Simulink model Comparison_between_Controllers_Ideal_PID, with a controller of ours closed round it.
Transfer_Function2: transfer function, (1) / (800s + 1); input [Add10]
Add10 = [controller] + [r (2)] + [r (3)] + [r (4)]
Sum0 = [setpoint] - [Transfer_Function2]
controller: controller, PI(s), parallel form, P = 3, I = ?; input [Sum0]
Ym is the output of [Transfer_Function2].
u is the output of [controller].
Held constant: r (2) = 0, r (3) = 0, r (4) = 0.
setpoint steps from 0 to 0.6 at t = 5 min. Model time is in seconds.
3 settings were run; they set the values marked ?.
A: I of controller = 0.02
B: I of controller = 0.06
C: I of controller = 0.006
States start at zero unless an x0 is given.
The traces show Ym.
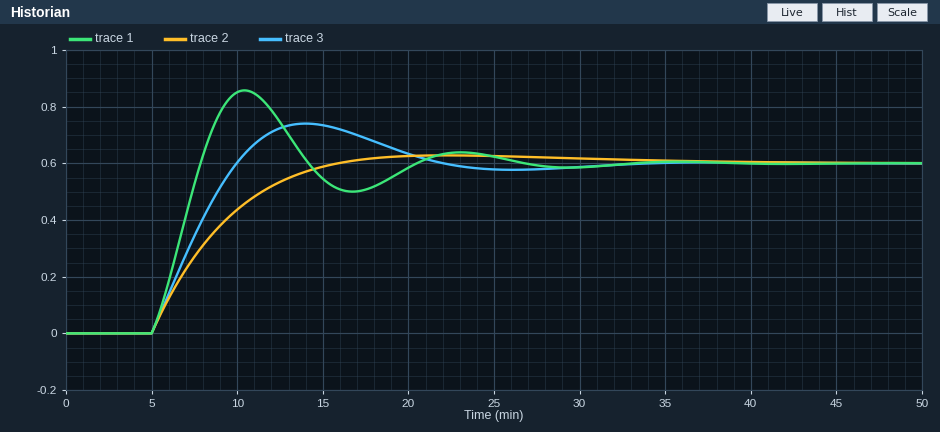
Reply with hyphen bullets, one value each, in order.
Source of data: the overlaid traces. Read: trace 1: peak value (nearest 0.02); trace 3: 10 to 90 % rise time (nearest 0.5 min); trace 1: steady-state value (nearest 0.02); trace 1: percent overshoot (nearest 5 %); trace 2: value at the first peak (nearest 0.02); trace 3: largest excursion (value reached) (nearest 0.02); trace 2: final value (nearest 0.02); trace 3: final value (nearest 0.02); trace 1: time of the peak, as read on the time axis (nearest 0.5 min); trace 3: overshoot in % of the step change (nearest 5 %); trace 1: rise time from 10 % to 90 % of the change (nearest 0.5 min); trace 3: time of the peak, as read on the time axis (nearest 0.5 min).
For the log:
- 0.86
- 4.0 min
- 0.60
- 45 %
- 0.62
- 0.74
- 0.60
- 0.60
- 10.5 min
- 25 %
- 2.0 min
- 14.0 min
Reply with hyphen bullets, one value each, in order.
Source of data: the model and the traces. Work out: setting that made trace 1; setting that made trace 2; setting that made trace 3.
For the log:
- B
- C
- A
